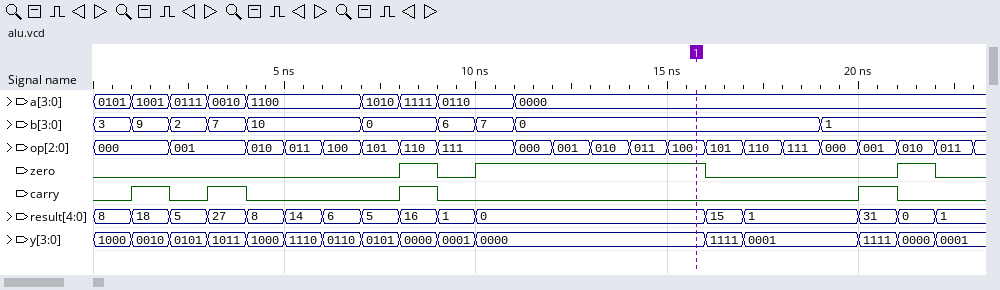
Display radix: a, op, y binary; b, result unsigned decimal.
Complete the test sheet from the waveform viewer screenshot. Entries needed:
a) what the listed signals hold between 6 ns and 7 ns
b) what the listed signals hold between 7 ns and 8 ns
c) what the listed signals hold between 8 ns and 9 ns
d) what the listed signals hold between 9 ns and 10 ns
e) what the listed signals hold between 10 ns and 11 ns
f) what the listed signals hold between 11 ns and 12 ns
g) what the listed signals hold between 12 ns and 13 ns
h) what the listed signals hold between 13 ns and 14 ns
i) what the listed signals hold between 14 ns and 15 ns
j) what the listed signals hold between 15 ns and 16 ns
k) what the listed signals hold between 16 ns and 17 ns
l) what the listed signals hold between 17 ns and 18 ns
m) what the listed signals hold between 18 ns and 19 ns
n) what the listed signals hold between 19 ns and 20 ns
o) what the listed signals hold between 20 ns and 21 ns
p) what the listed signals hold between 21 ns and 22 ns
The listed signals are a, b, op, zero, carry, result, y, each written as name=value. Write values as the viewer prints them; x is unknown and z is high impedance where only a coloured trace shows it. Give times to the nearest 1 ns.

a=1100, b=10, op=100, zero=0, carry=0, result=6, y=0110
a=1010, b=0, op=101, zero=0, carry=0, result=5, y=0101
a=1111, b=0, op=110, zero=1, carry=1, result=16, y=0000
a=0110, b=6, op=111, zero=0, carry=0, result=1, y=0001
a=0110, b=7, op=111, zero=1, carry=0, result=0, y=0000
a=0000, b=0, op=000, zero=1, carry=0, result=0, y=0000
a=0000, b=0, op=001, zero=1, carry=0, result=0, y=0000
a=0000, b=0, op=010, zero=1, carry=0, result=0, y=0000
a=0000, b=0, op=011, zero=1, carry=0, result=0, y=0000
a=0000, b=0, op=100, zero=1, carry=0, result=0, y=0000
a=0000, b=0, op=101, zero=0, carry=0, result=15, y=1111
a=0000, b=0, op=110, zero=0, carry=0, result=1, y=0001
a=0000, b=0, op=111, zero=0, carry=0, result=1, y=0001
a=0000, b=1, op=000, zero=0, carry=0, result=1, y=0001
a=0000, b=1, op=001, zero=0, carry=1, result=31, y=1111
a=0000, b=1, op=010, zero=1, carry=0, result=0, y=0000
